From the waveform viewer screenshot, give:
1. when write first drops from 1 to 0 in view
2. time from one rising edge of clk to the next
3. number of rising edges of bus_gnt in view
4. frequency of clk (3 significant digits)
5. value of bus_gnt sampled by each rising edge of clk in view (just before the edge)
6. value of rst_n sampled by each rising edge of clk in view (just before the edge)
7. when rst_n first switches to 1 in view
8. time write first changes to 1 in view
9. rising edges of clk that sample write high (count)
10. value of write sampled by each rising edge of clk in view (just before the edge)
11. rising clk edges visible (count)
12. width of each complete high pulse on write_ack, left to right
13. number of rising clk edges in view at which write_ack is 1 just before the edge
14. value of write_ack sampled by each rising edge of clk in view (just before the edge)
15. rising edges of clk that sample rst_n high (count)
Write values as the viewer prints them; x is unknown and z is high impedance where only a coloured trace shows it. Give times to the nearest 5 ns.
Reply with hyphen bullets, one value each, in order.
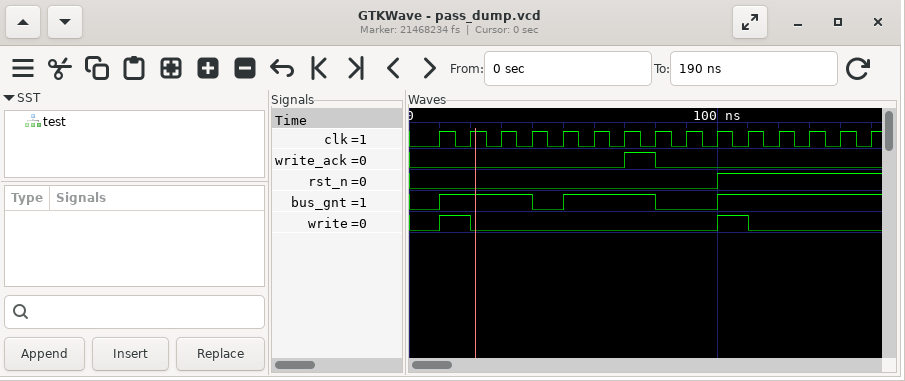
- 20 ns
- 10 ns
- 3
- 100 MHz
- 0 1 1 1 0 1 1 1 0 0 1 1 1 1 1
- 0 0 0 0 0 0 0 0 0 0 1 1 1 1 1
- 100 ns
- 10 ns
- 2
- 0 1 0 0 0 0 0 0 0 0 1 0 0 0 0
- 15
- 10 ns
- 1
- 0 0 0 0 0 0 0 1 0 0 0 0 0 0 0
- 5
